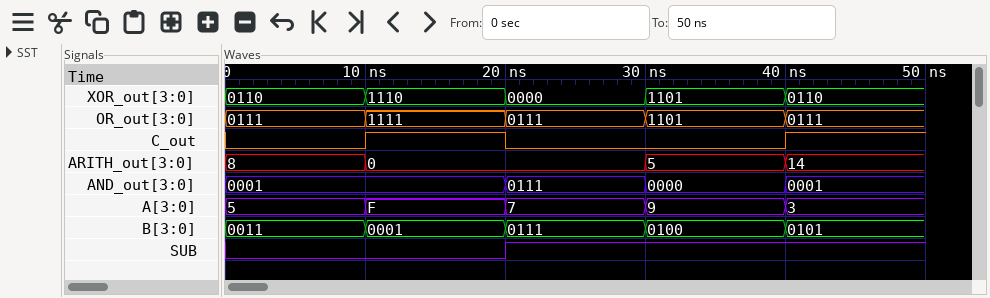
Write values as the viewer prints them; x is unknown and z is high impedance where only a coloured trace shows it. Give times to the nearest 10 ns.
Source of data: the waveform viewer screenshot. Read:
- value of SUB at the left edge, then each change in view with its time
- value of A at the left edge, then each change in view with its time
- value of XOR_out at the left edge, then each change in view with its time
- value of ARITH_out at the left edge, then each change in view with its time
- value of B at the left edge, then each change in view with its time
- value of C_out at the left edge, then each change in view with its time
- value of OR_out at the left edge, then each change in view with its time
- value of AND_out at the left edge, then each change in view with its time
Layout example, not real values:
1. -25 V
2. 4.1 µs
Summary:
1. 0, 1 at 20 ns
2. 5, F at 10 ns, 7 at 20 ns, 9 at 30 ns, 3 at 40 ns
3. 0110, 1110 at 10 ns, 0000 at 20 ns, 1101 at 30 ns, 0110 at 40 ns
4. 8, 0 at 10 ns, 5 at 30 ns, 14 at 40 ns
5. 0011, 0001 at 10 ns, 0111 at 20 ns, 0100 at 30 ns, 0101 at 40 ns
6. 0, 1 at 10 ns, 0 at 20 ns, 1 at 40 ns
7. 0111, 1111 at 10 ns, 0111 at 20 ns, 1101 at 30 ns, 0111 at 40 ns
8. 0001, 0111 at 20 ns, 0000 at 30 ns, 0001 at 40 ns
